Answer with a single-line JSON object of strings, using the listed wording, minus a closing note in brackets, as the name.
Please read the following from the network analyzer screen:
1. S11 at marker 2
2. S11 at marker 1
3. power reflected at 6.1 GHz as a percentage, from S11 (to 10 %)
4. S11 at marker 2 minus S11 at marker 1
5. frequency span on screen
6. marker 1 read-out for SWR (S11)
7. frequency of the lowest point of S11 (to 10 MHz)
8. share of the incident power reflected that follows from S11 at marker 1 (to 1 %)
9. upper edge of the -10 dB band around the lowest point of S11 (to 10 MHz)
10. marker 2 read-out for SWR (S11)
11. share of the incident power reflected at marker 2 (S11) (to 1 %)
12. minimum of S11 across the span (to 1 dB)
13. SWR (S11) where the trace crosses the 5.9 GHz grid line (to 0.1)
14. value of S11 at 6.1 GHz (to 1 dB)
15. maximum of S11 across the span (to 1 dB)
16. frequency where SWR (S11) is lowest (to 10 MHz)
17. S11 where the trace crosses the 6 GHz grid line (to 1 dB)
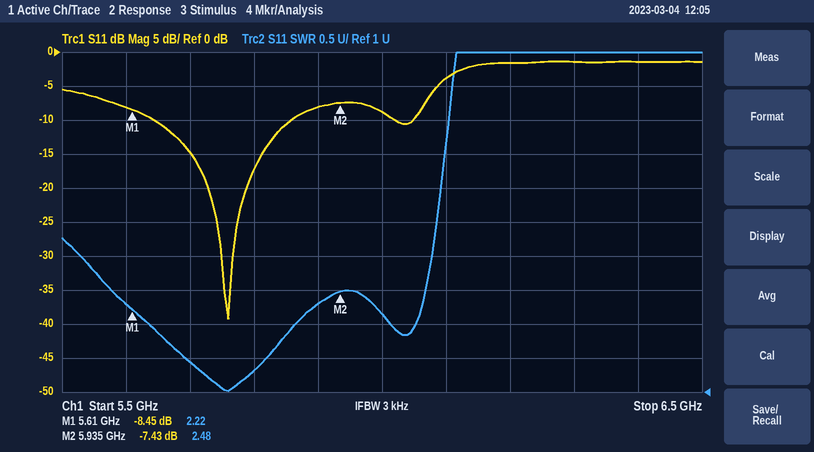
{"S11 at marker 2": "-7.43 dB", "S11 at marker 1": "-8.45 dB", "power reflected at 6.1 GHz as a percentage, from S11": "40 %", "S11 at marker 2 minus S11 at marker 1": "1.02 dB", "frequency span on screen": "1 GHz", "marker 1 read-out for SWR": "2.22", "frequency of the lowest point of S11": "5.76 GHz", "share of the incident power reflected that follows from S11 at marker 1": "14 %", "upper edge of the -10 dB band around the lowest point of S11": "5.86 GHz", "marker 2 read-out for SWR": "2.48", "share of the incident power reflected at marker 2 (S11)": "18 %", "minimum of S11 across the span": "-39 dB", "SWR (S11) where the trace crosses the 5.9 GHz grid line": "2.3", "value of S11 at 6.1 GHz": "-4 dB", "maximum of S11 across the span": "-1 dB", "frequency where SWR (S11) is lowest": "5.76 GHz", "S11 where the trace crosses the 6 GHz grid line": "-9 dB"}
